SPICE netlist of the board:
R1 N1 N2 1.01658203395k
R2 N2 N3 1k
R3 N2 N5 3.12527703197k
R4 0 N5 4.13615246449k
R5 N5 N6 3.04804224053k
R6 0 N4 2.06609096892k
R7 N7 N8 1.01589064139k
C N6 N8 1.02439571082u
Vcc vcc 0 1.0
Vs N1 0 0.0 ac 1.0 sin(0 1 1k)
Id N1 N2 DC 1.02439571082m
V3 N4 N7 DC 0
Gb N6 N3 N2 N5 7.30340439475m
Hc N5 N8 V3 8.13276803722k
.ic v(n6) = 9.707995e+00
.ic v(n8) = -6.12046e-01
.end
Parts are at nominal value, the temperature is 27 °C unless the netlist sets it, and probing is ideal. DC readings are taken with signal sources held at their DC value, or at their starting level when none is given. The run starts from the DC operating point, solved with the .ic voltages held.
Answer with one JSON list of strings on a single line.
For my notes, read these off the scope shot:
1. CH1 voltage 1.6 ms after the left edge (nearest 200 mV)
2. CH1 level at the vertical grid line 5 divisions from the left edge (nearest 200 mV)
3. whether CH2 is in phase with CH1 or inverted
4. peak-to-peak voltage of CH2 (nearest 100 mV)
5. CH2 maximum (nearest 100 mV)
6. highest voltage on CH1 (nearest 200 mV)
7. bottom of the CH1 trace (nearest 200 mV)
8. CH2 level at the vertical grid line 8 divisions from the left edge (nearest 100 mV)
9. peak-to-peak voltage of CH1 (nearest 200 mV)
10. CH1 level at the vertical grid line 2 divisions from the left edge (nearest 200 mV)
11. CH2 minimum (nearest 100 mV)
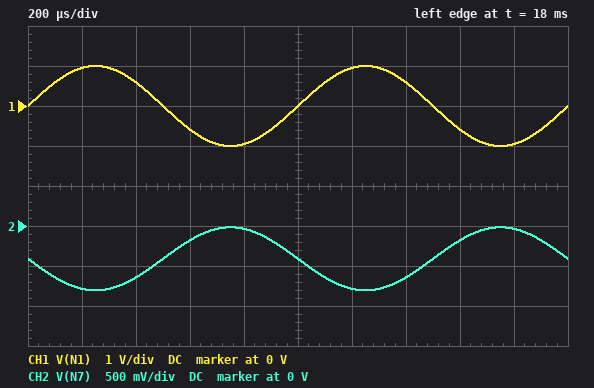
["-600 mV", "0 V", "inverted", "800 mV", "0 V", "1.0 V", "-1.0 V", "-200 mV", "2.0 V", "600 mV", "-800 mV"]
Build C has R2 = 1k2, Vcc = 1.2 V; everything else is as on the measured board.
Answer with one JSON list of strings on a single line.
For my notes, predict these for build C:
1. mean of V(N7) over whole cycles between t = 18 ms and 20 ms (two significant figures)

["-410 mV"]
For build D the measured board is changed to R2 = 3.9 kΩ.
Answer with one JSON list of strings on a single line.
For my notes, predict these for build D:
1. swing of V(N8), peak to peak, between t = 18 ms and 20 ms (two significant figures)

["1.2 V"]
